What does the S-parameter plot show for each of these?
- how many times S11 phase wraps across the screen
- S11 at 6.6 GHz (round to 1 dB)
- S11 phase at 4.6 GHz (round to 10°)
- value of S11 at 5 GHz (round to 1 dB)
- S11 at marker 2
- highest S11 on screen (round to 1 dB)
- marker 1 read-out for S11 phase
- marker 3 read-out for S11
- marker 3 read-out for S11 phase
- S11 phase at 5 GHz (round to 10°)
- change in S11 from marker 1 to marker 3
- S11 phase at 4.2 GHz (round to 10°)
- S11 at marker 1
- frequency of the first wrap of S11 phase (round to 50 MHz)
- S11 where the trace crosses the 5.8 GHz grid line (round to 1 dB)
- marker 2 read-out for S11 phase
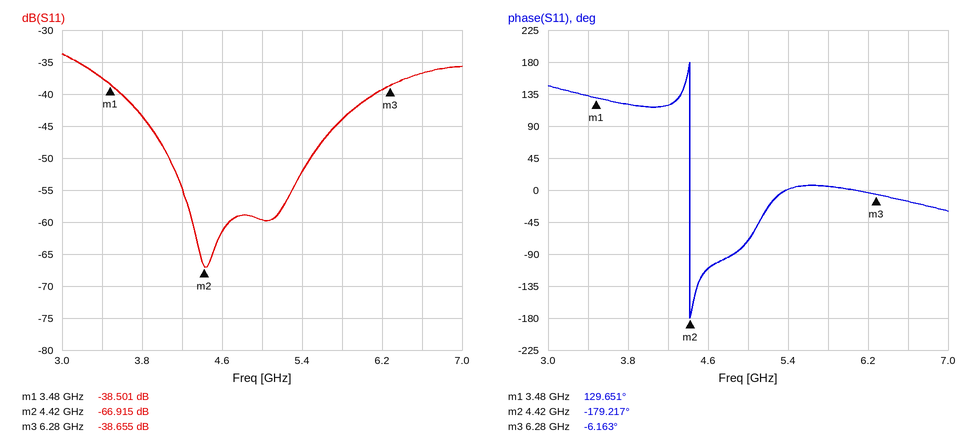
1
-37 dB
-110°
-60 dB
-66.915 dB
-34 dB
129.651°
-38.655 dB
-6.163°
-70°
-0.154 dB
120°
-38.501 dB
4.40 GHz
-44 dB
-179.217°
